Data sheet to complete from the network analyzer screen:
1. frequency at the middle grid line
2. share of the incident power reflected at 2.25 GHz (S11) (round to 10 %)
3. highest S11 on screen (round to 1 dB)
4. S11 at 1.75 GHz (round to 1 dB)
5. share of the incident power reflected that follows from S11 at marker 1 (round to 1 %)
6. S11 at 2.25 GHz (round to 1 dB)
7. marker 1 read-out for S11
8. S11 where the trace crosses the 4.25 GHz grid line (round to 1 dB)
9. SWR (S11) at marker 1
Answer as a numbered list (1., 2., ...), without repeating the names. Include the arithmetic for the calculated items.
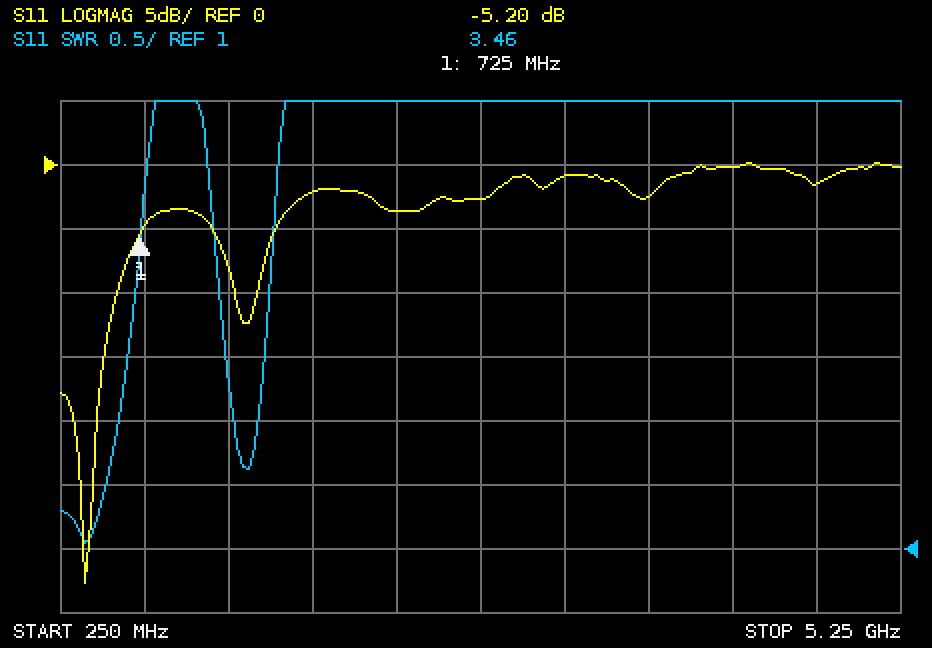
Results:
1. 2.75 GHz
2. 10^(-4/10) ≈ 40 %
3. 0 dB
4. -2 dB
5. 10^(-5.2/10) ≈ 30 %
6. -4 dB
7. -5.20 dB
8. 0 dB
9. 3.46
